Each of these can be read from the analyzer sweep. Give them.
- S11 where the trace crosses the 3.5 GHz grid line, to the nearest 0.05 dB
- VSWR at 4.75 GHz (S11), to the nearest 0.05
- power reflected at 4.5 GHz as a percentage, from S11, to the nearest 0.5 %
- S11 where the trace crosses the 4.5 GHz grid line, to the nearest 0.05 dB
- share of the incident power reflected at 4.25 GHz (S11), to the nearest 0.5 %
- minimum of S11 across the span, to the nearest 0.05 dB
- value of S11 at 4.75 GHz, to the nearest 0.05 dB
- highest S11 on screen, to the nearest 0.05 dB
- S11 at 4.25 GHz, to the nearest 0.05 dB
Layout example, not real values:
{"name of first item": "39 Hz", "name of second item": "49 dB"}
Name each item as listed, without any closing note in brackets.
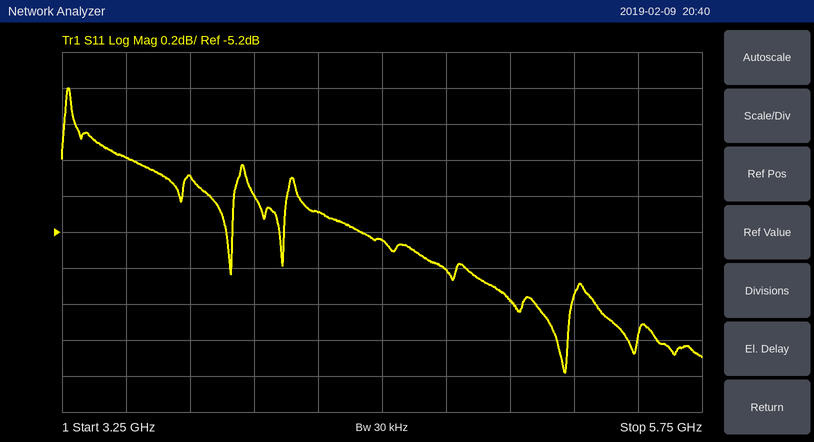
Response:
{"S11 where the trace crosses the 3.5 GHz grid line, to the nearest 0.05 dB": "-4.80 dB", "VSWR at 4.75 GHz (S11), to the nearest 0.05": "3.30", "power reflected at 4.5 GHz as a percentage, from S11, to the nearest 0.5 %": "30.0 %", "S11 where the trace crosses the 4.5 GHz grid line, to the nearest 0.05 dB": "-5.25 dB", "share of the incident power reflected at 4.25 GHz (S11), to the nearest 0.5 %": "31.0 %", "minimum of S11 across the span, to the nearest 0.05 dB": "-6.00 dB", "value of S11 at 4.75 GHz, to the nearest 0.05 dB": "-5.40 dB", "highest S11 on screen, to the nearest 0.05 dB": "-4.40 dB", "S11 at 4.25 GHz, to the nearest 0.05 dB": "-5.10 dB"}
